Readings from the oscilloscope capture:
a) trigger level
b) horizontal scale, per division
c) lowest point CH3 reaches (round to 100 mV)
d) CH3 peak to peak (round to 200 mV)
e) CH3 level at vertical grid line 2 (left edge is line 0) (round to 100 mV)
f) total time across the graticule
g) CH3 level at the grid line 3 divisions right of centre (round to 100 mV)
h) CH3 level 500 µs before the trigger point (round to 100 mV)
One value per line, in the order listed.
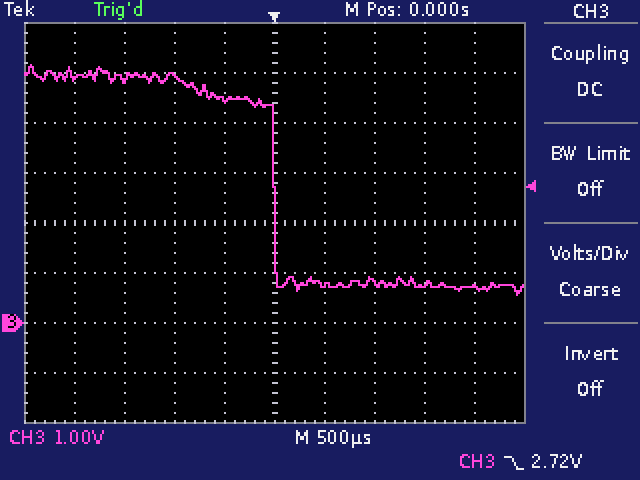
2.72 V
500 µs
600 mV
4.6 V
4.9 V
5 ms
800 mV
4.5 V
